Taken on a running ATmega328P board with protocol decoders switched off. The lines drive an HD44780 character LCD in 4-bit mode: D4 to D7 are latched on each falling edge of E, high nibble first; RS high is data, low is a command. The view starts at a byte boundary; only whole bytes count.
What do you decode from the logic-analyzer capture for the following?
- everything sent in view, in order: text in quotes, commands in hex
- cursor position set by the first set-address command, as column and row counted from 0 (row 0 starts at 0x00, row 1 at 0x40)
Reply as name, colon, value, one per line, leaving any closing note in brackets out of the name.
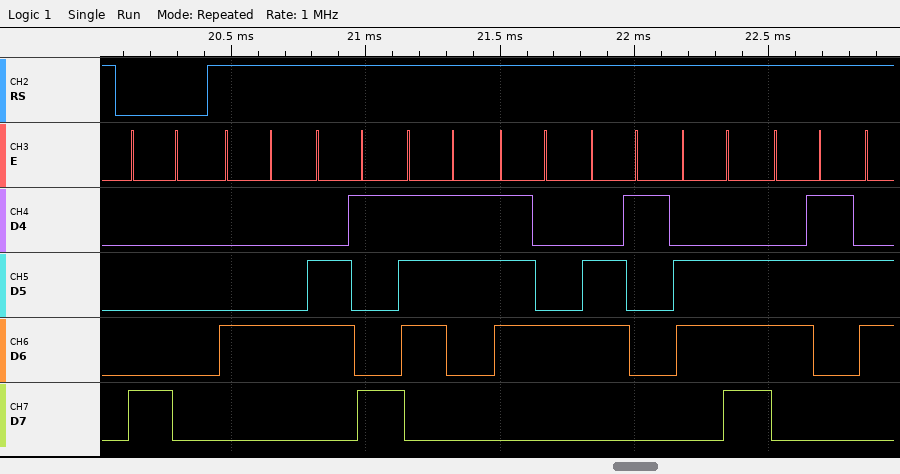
everything sent in view, in order: text in quotes, commands in hex: 0x80 "Distanc"
cursor position set by the first set-address command, as column and row counted from 0: column 0, row 0
